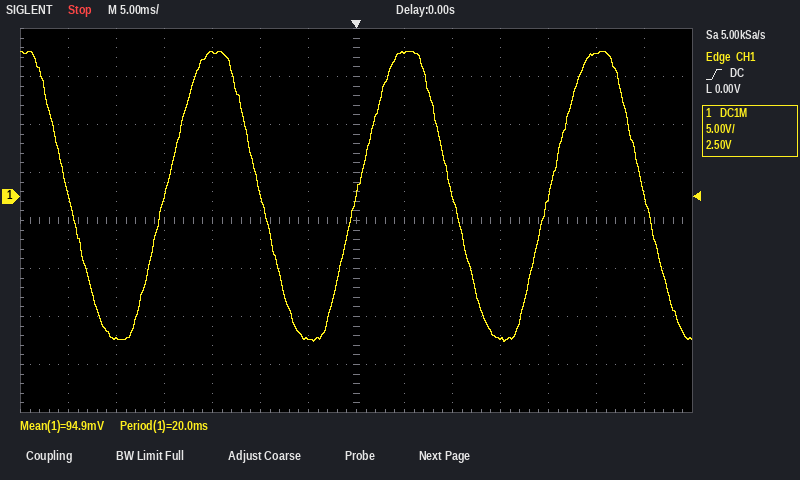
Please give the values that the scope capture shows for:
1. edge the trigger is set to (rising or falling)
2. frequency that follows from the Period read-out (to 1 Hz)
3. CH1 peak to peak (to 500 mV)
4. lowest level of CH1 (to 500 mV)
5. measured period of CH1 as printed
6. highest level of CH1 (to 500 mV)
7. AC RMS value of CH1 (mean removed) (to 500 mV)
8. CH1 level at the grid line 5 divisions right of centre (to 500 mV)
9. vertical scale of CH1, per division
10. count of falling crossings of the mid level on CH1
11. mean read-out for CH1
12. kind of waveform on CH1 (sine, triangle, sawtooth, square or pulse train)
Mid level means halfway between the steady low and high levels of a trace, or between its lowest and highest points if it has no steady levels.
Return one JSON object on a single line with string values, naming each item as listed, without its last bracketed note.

{"edge the trigger is set to": "rising", "frequency that follows from the Period read-out": "50 Hz", "CH1 peak to peak": "30.0 V", "lowest level of CH1": "-15.0 V", "measured period of CH1 as printed": "20.0 ms", "highest level of CH1": "15.0 V", "AC RMS value of CH1 (mean removed)": "10.5 V", "CH1 level at the grid line 5 divisions right of centre": "15.0 V", "vertical scale of CH1, per division": "5 V", "count of falling crossings of the mid level on CH1": "4", "mean read-out for CH1": "94.9 mV", "kind of waveform on CH1": "sine"}
